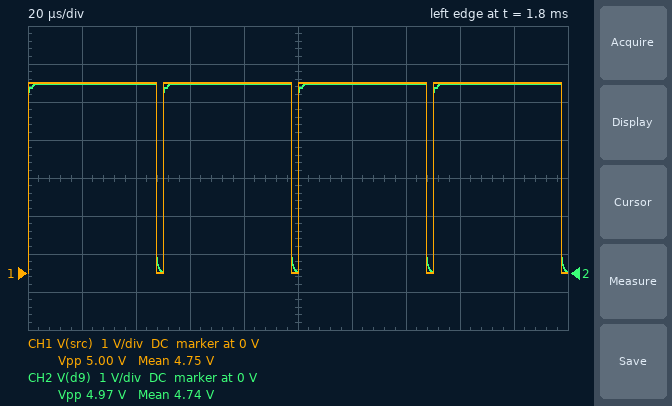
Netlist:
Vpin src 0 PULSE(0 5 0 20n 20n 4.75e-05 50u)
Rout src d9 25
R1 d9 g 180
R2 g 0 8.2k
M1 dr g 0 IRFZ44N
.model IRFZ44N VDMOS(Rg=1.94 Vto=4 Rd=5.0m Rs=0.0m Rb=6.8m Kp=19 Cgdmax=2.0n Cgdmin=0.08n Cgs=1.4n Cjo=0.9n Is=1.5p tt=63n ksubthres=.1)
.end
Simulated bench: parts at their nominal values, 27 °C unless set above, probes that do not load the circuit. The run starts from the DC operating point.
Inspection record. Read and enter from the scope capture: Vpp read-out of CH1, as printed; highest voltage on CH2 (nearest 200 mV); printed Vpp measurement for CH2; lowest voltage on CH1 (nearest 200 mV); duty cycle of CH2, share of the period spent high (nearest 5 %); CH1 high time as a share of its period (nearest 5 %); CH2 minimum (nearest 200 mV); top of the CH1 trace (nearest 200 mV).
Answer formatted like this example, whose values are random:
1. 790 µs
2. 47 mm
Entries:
1. 5.00 V
2. 5.0 V
3. 4.97 V
4. 0 V
5. 95 %
6. 95 %
7. 0 V
8. 5.0 V
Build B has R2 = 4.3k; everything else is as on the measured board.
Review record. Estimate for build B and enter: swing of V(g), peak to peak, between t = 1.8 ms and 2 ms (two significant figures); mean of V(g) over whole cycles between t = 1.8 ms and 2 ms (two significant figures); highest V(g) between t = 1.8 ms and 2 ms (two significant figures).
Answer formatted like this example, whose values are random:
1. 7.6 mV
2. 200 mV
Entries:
1. 4.7 V
2. 4.5 V
3. 4.8 V
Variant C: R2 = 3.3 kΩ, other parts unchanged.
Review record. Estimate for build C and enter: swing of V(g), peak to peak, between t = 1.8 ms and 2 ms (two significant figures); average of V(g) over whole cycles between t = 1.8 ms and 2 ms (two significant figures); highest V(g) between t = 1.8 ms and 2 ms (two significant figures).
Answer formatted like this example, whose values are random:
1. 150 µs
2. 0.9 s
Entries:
1. 4.6 V
2. 4.5 V
3. 4.7 V
